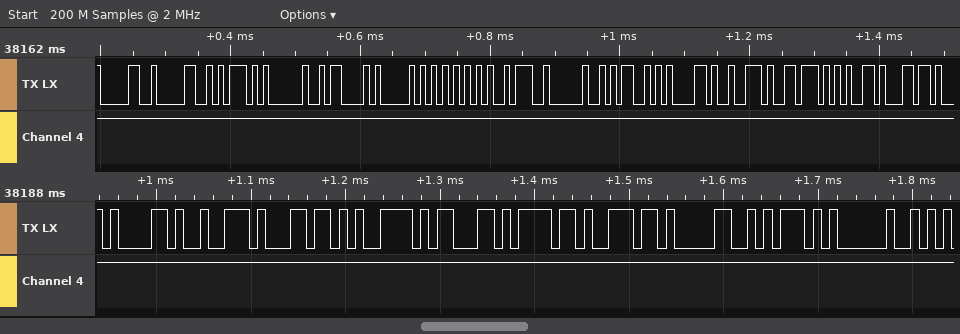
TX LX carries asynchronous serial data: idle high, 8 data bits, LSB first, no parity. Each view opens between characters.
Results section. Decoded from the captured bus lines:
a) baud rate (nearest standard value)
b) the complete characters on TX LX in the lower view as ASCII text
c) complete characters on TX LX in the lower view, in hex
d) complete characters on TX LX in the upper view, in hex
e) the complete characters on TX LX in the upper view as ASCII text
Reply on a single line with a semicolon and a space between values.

115200 baud; "arlycon0] "; 61, 72, 6C, 79, 63, 6F, 6E, 30, 5D, 20; 30, 30, 5D, 20, 43, 50, 55, 3A, 20, 4D, 61, 72, 76, 65, 6C; "00] CPU: Marvel"
